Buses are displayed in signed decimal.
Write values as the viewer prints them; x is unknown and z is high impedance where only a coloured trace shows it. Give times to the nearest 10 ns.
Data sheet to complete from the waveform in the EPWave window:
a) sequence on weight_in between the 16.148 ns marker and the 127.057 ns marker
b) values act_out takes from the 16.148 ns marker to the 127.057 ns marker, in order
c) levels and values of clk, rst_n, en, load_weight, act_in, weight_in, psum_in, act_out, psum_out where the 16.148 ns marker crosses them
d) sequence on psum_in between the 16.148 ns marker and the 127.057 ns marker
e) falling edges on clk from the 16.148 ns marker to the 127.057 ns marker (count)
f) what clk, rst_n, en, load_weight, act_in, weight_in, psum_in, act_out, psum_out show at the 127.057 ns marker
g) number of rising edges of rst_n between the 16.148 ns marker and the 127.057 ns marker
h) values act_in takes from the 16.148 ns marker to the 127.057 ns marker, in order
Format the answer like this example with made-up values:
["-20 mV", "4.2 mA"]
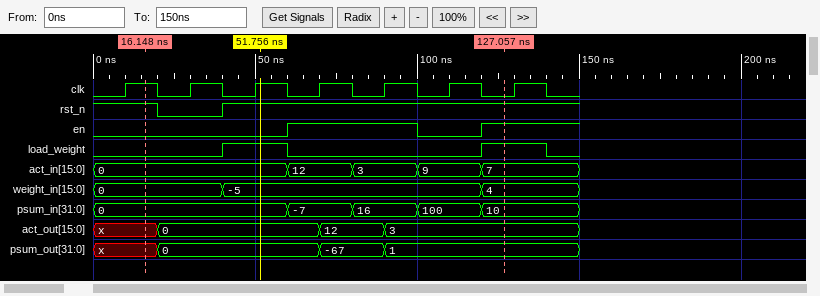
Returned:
["0, -5, 4", "x, 0, 12, 3", "clk=1, rst_n=1, en=0, load_weight=0, act_in=0, weight_in=0, psum_in=0, act_out=x, psum_out=x", "0, -7, 16, 100, 10", "6", "clk=0, rst_n=1, en=1, load_weight=1, act_in=7, weight_in=4, psum_in=10, act_out=3, psum_out=1", "1", "0, 12, 3, 9, 7"]
